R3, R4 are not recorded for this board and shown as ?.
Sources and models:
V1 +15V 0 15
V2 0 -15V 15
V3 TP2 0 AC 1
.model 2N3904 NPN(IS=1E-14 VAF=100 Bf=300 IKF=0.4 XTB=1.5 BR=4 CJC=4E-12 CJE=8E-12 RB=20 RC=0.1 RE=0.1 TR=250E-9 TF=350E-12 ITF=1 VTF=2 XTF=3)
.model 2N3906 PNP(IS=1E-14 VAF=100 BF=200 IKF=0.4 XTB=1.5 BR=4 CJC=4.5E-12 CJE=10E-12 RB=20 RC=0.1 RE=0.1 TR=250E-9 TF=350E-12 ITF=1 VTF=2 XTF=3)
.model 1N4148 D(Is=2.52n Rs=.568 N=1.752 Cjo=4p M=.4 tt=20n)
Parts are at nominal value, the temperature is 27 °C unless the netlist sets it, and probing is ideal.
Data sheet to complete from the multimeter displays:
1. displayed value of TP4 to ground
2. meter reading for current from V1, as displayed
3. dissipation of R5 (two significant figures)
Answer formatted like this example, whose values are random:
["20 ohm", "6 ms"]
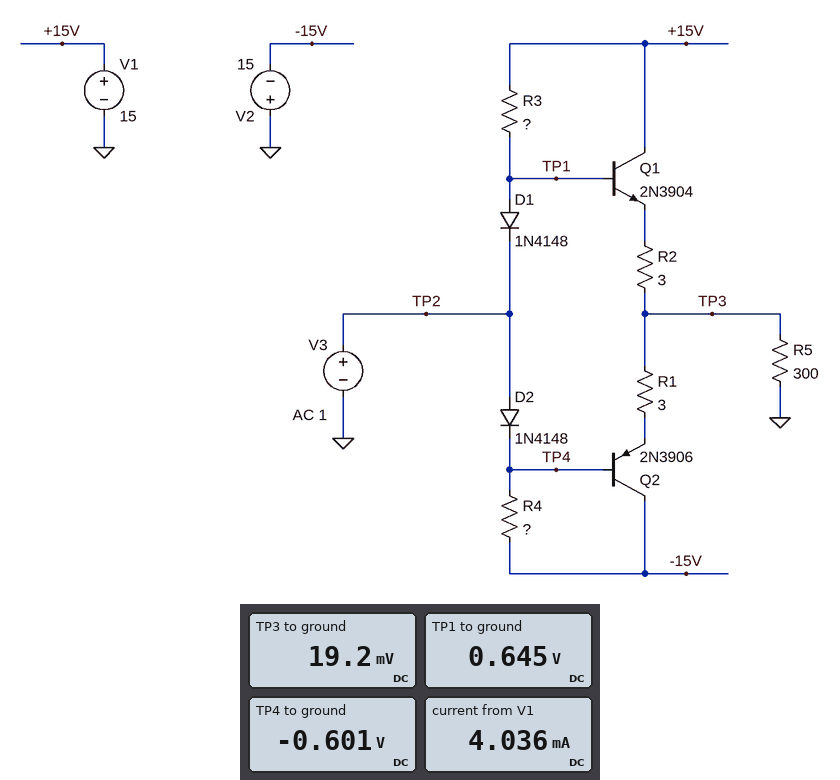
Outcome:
["-0.601 V", "4.036 mA", "1.2 µW"]
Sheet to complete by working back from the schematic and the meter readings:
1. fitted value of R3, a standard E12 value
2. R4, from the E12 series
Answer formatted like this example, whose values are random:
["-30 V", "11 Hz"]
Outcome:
["3.9 kΩ", "10 kΩ"]
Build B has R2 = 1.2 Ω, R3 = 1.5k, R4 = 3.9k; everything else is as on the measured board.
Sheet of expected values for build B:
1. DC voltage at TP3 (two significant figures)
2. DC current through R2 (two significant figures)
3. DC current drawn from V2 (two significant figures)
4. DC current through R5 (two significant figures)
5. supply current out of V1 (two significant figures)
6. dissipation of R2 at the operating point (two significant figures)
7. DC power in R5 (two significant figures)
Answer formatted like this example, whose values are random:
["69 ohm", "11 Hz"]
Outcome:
["24 mV", "1.7 mA", "5.3 mA", "80 µA", "11 mA", "3.5 µW", "1.9 µW"]
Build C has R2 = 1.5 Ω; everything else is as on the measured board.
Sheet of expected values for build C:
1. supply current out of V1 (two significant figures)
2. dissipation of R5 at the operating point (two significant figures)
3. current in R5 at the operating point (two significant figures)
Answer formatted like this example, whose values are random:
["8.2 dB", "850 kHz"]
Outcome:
["4.0 mA", "1.3 µW", "65 µA"]
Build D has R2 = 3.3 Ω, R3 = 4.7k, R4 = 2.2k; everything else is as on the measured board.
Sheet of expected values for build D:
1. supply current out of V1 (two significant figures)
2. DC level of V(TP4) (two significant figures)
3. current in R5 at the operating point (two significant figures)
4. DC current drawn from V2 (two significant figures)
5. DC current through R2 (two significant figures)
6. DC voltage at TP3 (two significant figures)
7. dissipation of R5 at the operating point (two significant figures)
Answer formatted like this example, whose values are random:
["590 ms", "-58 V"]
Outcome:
["4.0 mA", "-670 mV", "58 µA", "7.5 mA", "960 µA", "-17 mV", "1.0 µW"]
